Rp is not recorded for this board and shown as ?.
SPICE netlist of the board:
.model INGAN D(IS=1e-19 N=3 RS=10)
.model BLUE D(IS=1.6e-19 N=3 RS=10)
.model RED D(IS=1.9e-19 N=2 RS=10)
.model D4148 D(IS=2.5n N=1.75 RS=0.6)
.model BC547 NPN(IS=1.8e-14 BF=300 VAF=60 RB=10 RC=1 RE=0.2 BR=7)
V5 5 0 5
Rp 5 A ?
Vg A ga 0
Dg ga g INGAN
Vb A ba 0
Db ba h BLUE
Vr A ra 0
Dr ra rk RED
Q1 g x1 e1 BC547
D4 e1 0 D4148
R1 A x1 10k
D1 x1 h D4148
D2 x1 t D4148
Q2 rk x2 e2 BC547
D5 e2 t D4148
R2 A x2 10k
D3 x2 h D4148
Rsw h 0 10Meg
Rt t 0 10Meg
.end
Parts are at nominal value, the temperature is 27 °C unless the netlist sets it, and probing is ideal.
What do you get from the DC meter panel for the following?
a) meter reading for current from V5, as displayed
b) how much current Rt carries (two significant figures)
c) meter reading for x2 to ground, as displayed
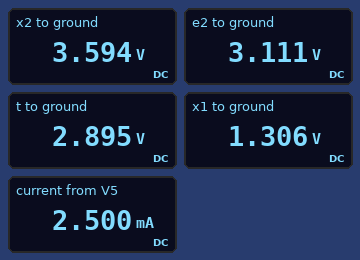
2.500 mA
290 nA
3.594 V
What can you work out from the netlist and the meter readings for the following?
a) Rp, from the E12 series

560 Ω
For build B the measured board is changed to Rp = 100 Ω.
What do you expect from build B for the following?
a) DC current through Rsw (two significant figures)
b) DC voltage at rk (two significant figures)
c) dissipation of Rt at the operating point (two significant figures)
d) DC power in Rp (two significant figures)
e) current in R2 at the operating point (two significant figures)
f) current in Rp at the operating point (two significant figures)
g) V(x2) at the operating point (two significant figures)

370 nA
3.4 V
1.0 µW
12 mW
690 nA
11 mA
3.9 V
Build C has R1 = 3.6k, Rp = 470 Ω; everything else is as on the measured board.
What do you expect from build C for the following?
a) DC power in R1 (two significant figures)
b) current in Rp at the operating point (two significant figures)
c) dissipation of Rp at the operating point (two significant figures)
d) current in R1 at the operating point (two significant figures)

1.4 mW
3.0 mA
4.2 mW
630 µA
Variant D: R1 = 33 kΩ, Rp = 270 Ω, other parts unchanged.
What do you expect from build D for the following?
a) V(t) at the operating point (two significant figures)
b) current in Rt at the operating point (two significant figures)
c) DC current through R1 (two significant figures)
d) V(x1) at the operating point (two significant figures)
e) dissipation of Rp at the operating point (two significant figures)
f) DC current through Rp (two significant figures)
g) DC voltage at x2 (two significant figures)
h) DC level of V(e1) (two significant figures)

3.0 V
300 nA
73 µA
1.3 V
5.8 mW
4.6 mA
3.7 V
660 mV
